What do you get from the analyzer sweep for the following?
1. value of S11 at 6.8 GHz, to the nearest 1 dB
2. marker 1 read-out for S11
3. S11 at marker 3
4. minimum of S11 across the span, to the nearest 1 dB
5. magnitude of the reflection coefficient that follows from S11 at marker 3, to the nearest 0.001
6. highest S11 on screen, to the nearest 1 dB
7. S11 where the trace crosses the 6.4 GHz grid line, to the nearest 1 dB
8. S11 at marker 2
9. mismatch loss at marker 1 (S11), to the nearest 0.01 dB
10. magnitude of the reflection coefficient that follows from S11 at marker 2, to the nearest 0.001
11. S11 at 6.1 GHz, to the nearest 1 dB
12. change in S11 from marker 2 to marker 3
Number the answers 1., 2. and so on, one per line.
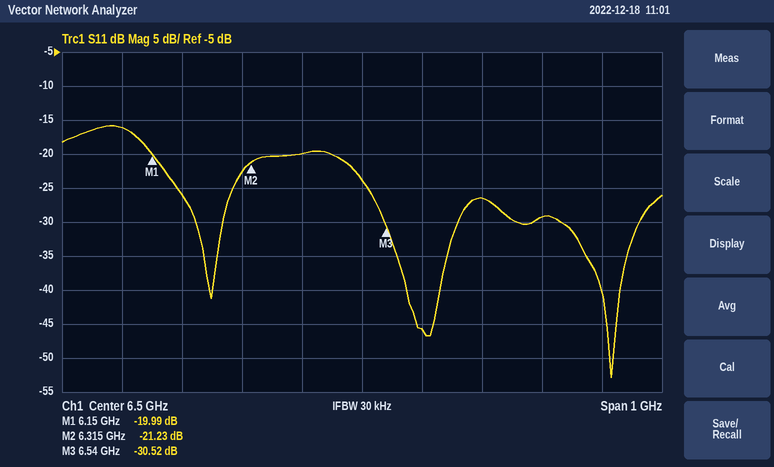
1. -29 dB
2. -19.99 dB
3. -30.52 dB
4. -53 dB
5. 0.030
6. -16 dB
7. -20 dB
8. -21.23 dB
9. 0.04 dB
10. 0.087
11. -16 dB
12. -9.29 dB
